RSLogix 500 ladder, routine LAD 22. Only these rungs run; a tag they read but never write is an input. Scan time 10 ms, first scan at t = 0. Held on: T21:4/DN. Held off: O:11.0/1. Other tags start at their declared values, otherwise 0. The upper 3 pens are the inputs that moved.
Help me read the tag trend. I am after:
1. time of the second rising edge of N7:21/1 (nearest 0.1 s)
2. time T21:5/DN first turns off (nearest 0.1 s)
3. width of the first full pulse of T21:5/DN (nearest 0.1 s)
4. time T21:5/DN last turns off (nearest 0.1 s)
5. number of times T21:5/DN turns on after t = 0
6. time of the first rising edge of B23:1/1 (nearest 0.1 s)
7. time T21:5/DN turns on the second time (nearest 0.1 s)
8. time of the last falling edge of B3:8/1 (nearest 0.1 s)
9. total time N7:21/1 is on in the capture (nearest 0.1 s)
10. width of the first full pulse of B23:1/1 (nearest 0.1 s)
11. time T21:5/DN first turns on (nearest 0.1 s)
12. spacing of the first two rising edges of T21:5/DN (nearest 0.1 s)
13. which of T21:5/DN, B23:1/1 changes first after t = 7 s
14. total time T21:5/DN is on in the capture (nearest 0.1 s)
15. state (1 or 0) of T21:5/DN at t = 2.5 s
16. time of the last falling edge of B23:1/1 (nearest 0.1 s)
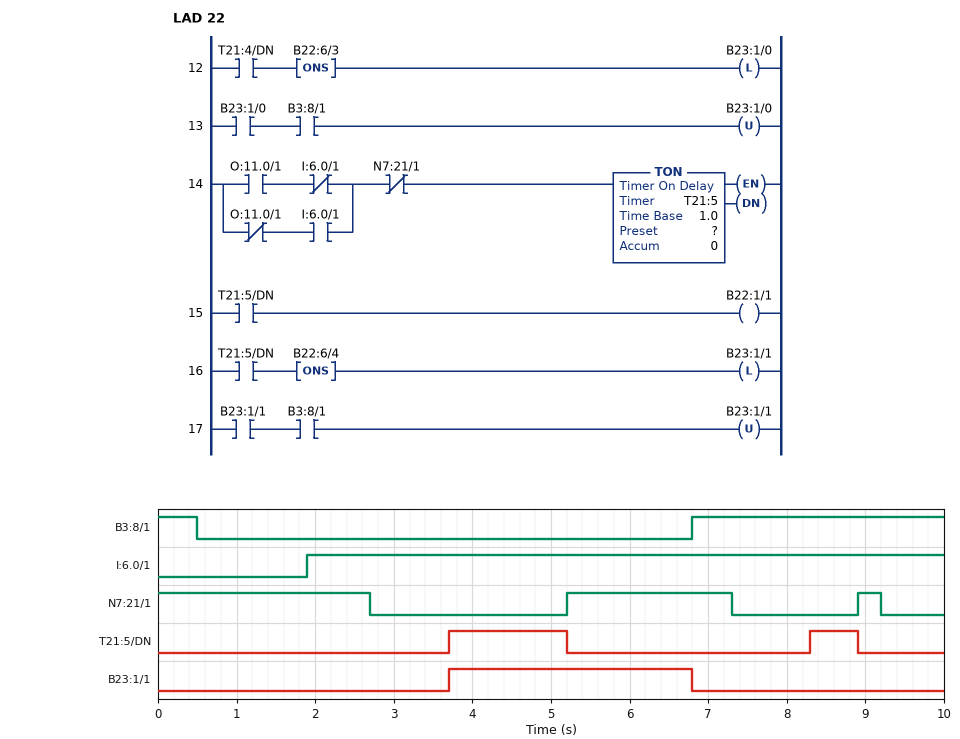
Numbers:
8.9 s
5.2 s
1.5 s
8.9 s
2
3.7 s
8.3 s
0.5 s
5.1 s
3.1 s
3.7 s
4.6 s
T21:5/DN
2.1 s
0
6.8 s
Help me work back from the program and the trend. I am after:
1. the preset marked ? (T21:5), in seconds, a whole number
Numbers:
1 s
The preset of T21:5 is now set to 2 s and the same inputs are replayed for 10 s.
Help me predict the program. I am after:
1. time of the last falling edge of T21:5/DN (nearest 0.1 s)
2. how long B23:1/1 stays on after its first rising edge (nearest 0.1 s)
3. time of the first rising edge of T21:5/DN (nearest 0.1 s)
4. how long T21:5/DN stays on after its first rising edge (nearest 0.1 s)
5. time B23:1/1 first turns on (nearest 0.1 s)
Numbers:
5.2 s
2.1 s
4.7 s
0.5 s
4.7 s
